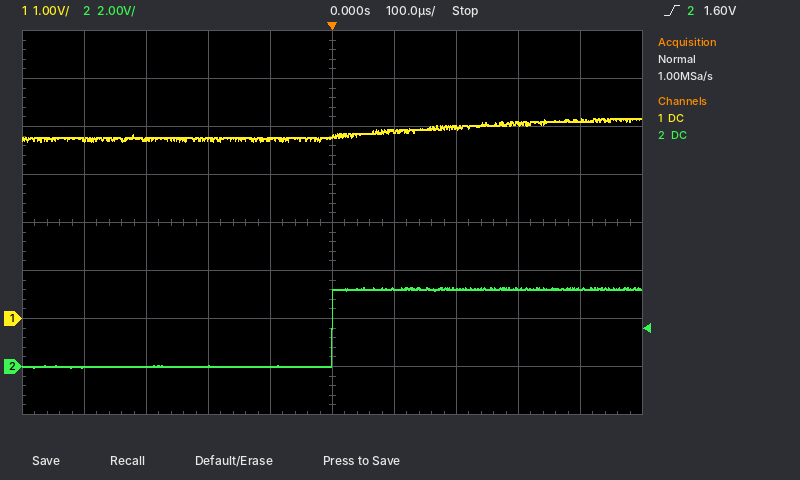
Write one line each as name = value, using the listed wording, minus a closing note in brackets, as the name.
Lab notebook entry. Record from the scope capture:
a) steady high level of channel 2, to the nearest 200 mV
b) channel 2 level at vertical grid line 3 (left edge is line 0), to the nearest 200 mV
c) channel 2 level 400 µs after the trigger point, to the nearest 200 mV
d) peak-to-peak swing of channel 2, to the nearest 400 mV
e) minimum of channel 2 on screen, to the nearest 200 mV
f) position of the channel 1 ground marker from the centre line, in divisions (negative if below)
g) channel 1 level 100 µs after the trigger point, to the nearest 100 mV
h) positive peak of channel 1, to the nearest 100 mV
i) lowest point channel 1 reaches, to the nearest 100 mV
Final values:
steady high level of channel 2, to the nearest 200 mV = 3.2 V
channel 2 level at vertical grid line 3 (left edge is line 0), to the nearest 200 mV = 0.0 V
channel 2 level 400 µs after the trigger point, to the nearest 200 mV = 3.2 V
peak-to-peak swing of channel 2, to the nearest 400 mV = 3.2 V
minimum of channel 2 on screen, to the nearest 200 mV = 0.0 V
position of the channel 1 ground marker from the centre line, in divisions = -2.0 div
channel 1 level 100 µs after the trigger point, to the nearest 100 mV = 3.9 V
positive peak of channel 1, to the nearest 100 mV = 4.2 V
lowest point channel 1 reaches, to the nearest 100 mV = 3.7 V
